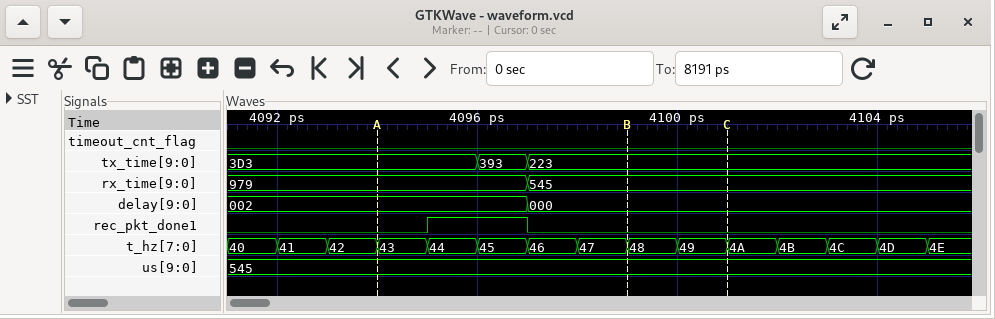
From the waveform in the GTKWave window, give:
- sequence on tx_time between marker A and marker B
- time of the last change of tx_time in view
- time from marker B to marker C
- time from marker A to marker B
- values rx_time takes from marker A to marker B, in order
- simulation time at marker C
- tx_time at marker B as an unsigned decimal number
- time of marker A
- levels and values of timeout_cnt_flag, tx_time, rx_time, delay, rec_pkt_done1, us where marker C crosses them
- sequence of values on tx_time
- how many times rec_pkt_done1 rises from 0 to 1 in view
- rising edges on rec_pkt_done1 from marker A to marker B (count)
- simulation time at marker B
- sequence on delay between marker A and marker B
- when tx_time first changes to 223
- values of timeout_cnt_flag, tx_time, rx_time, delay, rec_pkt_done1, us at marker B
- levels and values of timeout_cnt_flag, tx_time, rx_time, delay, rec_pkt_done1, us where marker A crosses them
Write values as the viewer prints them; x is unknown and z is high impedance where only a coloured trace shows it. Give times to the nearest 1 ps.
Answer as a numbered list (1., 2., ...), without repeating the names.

1. 3D3, 393, 223
2. 4097 ps
3. 2 ps
4. 5 ps
5. 979, 545
6. 4101 ps
7. 547
8. 4094 ps
9. timeout_cnt_flag=0, tx_time=223, rx_time=545, delay=000, rec_pkt_done1=0, us=545
10. 3D3, 393, 223
11. 1
12. 1
13. 4099 ps
14. 002, 000
15. 4097 ps
16. timeout_cnt_flag=0, tx_time=223, rx_time=545, delay=000, rec_pkt_done1=0, us=545
17. timeout_cnt_flag=0, tx_time=3D3, rx_time=979, delay=002, rec_pkt_done1=0, us=545
